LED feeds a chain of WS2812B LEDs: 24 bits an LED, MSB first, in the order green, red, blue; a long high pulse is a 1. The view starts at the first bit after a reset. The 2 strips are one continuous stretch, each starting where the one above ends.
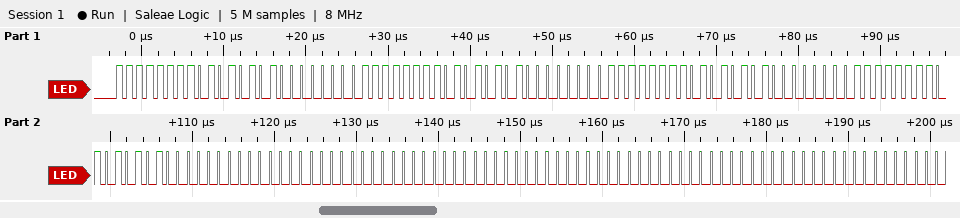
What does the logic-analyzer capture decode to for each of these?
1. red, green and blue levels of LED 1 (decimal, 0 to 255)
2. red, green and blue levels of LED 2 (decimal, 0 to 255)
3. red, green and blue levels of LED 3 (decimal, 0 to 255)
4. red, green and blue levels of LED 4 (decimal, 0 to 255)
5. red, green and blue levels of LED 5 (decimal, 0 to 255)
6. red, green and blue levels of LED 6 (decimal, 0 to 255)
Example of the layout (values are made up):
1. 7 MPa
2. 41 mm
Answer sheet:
1. 85, 255, 0
2. 85, 255, 0
3. 85, 255, 0
4. 85, 255, 0
5. 0, 0, 0
6. 0, 0, 0
